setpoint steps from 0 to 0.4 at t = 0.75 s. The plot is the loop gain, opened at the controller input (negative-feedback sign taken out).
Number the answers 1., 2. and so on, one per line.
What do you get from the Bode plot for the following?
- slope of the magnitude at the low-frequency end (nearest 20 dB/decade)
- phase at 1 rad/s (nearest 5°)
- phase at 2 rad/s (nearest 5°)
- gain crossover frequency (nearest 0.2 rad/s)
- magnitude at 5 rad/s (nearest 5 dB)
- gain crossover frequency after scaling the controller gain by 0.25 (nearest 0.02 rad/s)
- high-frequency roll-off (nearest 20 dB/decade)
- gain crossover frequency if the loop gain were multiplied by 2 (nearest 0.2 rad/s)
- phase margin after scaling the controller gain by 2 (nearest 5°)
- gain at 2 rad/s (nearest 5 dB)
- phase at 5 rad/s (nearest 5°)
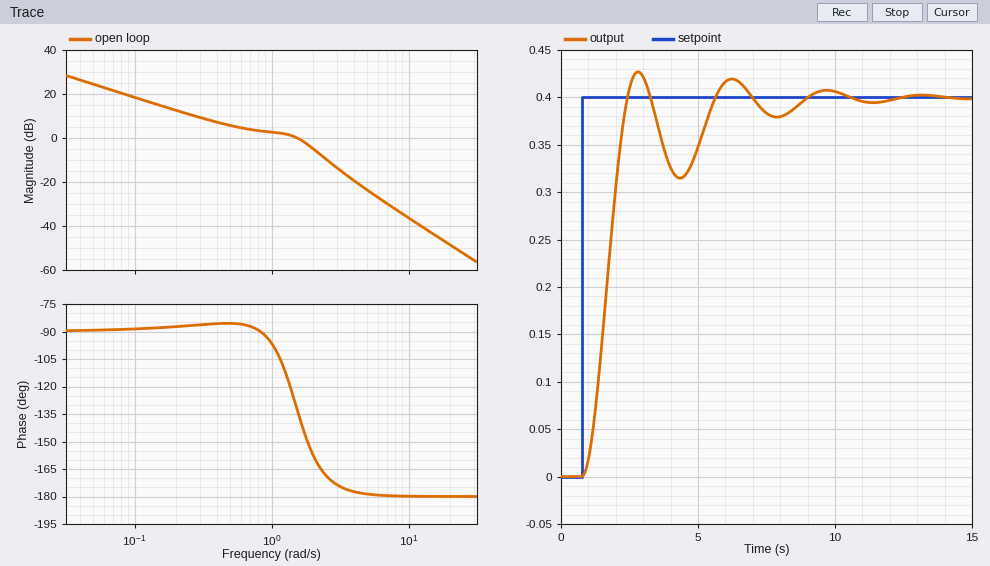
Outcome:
1. -20 dB/decade
2. -95°
3. -155°
4. 1.6 rad/s
5. -25 dB
6. 0.22 rad/s
7. -40 dB/decade
8. 2.2 rad/s
9. 20°
10. -5 dB
11. -180°
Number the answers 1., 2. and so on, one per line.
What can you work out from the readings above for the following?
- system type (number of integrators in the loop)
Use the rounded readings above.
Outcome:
1. 1
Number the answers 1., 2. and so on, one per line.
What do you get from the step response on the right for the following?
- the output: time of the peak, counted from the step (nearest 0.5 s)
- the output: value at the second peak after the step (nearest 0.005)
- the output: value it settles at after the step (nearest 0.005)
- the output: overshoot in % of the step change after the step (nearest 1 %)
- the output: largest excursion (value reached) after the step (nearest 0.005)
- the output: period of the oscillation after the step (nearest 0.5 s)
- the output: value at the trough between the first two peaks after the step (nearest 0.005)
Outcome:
1. 2.0 s
2. 0.420
3. 0.400
4. 7 %
5. 0.425
6. 3.5 s
7. 0.315
